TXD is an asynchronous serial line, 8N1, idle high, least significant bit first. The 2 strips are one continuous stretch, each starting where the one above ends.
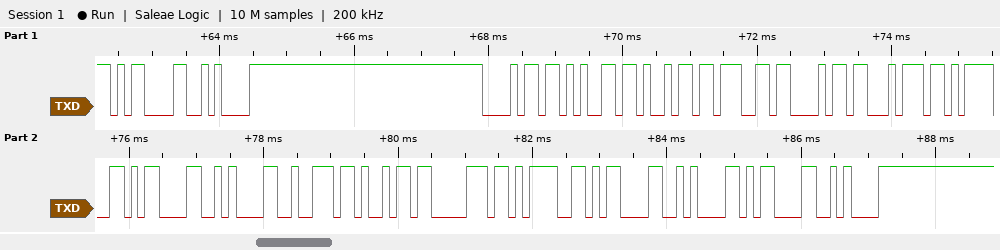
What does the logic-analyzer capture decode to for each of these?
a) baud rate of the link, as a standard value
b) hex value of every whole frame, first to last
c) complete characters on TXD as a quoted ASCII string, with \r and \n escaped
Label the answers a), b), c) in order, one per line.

a) 9600 baud
b) 0D 0A 68 65 69 67 68 74 3D 0D 0A 72 69 70 3D 0D 0A 0D 0A
c) "\r\nheight=\r\nrip=\r\n\r\n"
